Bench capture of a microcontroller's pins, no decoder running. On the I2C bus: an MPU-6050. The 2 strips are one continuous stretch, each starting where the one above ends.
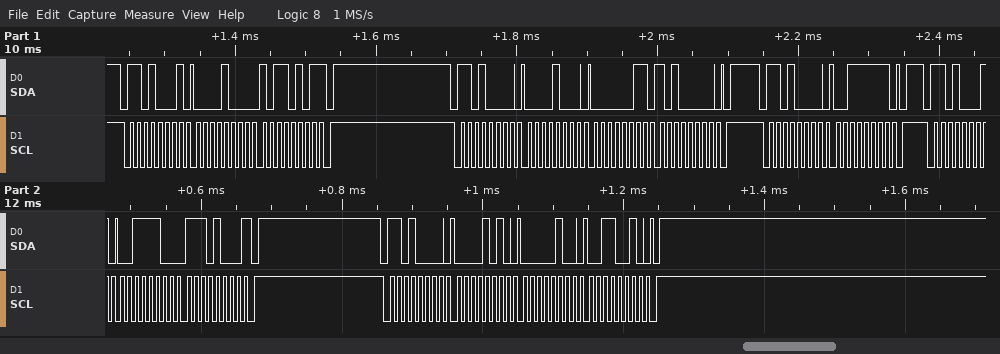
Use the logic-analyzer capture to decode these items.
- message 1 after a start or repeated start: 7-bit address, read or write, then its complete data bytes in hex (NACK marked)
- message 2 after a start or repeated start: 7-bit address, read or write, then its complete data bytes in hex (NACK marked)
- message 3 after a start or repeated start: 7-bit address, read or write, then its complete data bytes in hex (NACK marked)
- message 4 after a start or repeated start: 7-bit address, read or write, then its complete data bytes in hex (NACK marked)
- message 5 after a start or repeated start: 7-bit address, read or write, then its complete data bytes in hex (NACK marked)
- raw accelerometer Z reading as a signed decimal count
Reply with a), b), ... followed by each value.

a) 0x68 read: 08 B5 NACK
b) 0x68 write: 08 03 A0
c) 0x68 write: 3F
d) 0x68 read: 3C E8 NACK
e) 0x68 write: 0A 04 32
f) 15592
